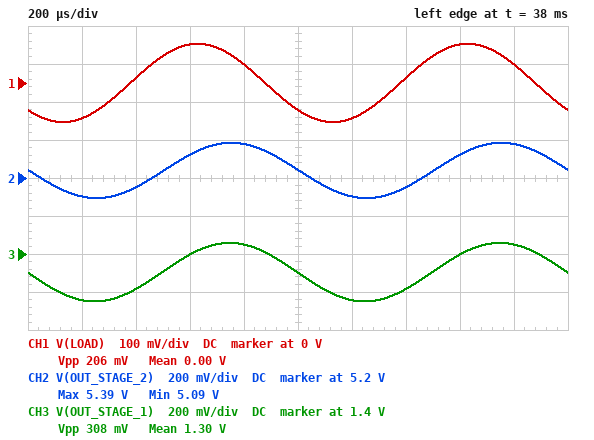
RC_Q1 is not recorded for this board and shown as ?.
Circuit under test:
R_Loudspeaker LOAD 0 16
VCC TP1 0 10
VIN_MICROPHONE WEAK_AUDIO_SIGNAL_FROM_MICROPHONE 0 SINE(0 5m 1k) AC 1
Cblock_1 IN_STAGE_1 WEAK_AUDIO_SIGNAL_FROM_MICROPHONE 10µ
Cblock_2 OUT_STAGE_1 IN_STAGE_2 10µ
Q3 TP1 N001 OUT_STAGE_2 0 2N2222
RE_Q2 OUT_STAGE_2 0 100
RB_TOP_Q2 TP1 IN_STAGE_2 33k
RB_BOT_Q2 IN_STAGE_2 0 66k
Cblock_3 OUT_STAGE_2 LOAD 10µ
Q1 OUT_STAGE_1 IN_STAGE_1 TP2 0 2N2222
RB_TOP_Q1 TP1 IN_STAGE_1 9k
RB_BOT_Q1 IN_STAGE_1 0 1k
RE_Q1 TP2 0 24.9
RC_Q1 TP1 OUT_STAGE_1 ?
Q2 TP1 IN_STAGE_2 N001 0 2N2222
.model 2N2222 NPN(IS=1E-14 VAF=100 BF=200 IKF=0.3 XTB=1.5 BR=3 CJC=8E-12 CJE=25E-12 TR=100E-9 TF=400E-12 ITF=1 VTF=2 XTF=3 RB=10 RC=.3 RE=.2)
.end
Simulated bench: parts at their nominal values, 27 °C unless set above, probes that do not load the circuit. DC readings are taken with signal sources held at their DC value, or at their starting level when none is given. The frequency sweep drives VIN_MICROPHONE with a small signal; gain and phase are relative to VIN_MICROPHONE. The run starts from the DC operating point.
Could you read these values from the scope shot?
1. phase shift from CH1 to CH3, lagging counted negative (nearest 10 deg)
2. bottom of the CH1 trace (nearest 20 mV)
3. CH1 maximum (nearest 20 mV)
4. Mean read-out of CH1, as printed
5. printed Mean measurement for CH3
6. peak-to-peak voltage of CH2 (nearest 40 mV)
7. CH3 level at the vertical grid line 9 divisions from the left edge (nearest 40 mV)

-40 deg
-100 mV
100 mV
0.00 V
1.30 V
280 mV
1.44 V
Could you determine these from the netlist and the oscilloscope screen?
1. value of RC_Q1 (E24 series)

910 Ω
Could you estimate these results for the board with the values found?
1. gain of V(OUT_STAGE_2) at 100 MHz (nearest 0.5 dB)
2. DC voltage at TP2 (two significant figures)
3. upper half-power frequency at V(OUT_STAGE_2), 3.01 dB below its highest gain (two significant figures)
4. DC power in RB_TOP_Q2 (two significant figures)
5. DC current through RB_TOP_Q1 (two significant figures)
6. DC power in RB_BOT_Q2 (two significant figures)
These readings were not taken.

-0.5 dB
240 mV
10 MHz
340 µW
1.0 mA
670 µW
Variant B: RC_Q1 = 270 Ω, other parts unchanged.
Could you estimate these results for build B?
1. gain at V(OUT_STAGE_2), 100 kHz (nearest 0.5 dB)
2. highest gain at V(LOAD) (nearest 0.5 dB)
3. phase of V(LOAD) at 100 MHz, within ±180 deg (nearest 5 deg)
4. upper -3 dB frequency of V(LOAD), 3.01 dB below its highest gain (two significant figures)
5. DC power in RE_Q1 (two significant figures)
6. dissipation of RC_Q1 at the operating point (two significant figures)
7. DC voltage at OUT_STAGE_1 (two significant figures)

18.5 dB
19.0 dB
65 deg
25 MHz
2.4 mW
25 mW
7.4 V
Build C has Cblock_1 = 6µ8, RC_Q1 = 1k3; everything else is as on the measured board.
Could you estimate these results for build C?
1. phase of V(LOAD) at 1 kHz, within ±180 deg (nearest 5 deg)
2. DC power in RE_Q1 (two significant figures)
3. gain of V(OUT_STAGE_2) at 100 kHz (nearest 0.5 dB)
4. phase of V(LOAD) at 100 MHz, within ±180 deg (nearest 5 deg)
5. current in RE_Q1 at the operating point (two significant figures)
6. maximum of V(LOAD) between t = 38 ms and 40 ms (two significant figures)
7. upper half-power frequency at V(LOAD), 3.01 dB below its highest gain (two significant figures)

-115 deg
1.4 mW
14.0 dB
-20 deg
7.6 mA
36 mV
790 kHz
